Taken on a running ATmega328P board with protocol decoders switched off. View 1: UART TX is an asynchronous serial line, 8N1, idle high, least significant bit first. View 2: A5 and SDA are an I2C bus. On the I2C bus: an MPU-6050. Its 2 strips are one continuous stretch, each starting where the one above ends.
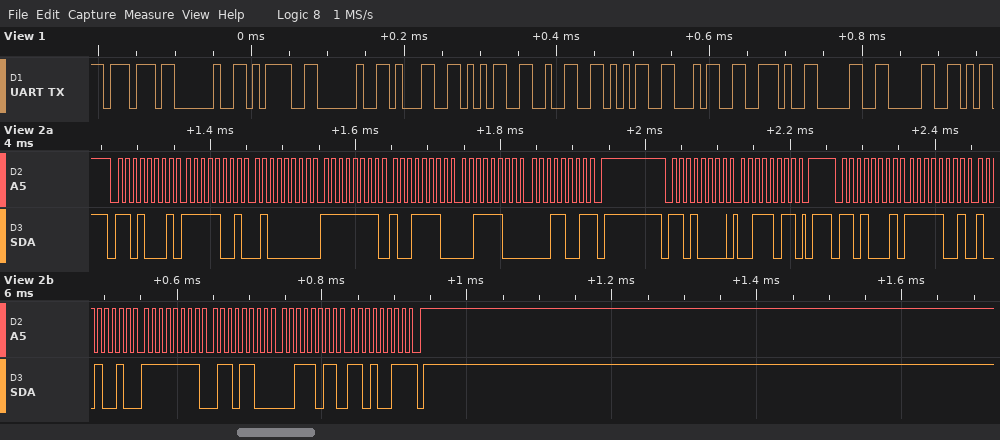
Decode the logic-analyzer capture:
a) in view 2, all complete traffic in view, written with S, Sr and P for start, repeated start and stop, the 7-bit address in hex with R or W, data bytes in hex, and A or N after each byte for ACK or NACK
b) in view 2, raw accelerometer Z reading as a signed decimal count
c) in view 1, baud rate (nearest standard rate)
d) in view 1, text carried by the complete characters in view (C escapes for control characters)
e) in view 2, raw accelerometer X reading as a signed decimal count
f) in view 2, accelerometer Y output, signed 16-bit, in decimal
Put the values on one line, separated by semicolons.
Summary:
S 68R A F9 A 40 A FF A 9E A 3C A 19 N P S 68W A 3B A P S 68R A F9 A 92 A FF A 6C A 3B A D3 N P; 15315; 115200 baud; "w = 15254.00"; -1646; -148
